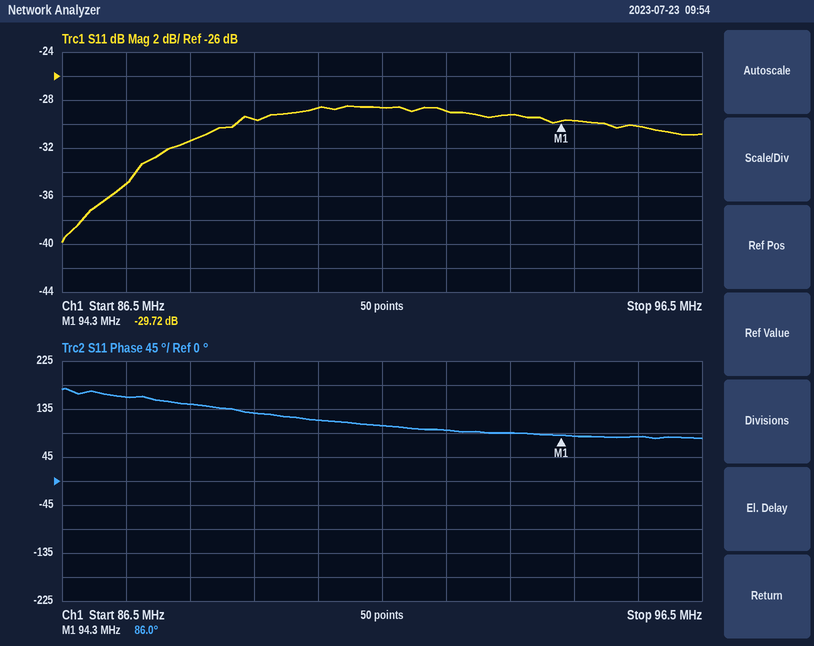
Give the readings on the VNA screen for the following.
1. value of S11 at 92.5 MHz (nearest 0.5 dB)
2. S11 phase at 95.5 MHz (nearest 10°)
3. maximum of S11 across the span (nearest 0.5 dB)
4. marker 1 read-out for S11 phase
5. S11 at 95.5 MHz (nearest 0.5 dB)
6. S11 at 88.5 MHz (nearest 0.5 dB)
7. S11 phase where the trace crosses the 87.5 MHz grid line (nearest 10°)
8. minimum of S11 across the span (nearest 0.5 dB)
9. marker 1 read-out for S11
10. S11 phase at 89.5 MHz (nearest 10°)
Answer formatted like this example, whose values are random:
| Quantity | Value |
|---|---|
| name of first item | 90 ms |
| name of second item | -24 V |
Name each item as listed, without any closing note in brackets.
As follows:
| Quantity | Value |
|---|---|
| value of S11 at 92.5 MHz | -29.0 dB |
| S11 phase at 95.5 MHz | 80° |
| maximum of S11 across the span | -28.5 dB |
| marker 1 read-out for S11 phase | 86.0° |
| S11 at 95.5 MHz | -30.0 dB |
| S11 at 88.5 MHz | -31.5 dB |
| S11 phase where the trace crosses the 87.5 MHz grid line | 160° |
| minimum of S11 across the span | -40.0 dB |
| marker 1 read-out for S11 | -29.72 dB |
| S11 phase at 89.5 MHz | 130° |
